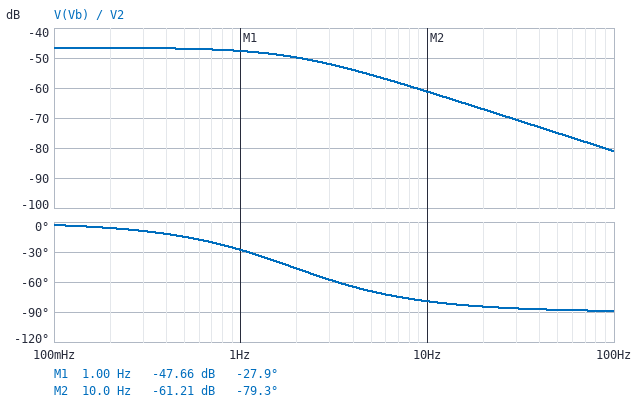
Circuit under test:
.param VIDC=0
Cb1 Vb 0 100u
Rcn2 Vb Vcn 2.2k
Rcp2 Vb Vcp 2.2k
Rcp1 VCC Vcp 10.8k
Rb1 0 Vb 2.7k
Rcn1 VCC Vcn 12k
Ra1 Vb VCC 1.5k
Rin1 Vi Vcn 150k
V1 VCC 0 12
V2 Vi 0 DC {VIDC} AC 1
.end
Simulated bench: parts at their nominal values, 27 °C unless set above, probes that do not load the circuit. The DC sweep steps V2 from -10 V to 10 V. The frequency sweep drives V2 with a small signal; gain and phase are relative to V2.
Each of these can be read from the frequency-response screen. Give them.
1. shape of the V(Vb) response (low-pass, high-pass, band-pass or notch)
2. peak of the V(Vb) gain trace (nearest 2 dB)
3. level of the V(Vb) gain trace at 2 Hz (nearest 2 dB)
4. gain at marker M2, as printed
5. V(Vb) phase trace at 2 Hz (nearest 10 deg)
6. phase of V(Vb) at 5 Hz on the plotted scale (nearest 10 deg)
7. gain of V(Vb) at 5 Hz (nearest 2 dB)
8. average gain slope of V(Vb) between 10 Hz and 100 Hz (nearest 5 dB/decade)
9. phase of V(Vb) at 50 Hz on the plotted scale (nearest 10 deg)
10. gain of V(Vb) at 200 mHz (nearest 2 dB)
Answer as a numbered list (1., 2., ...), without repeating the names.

1. low-pass
2. -46 dB
3. -50 dB
4. -61.21 dB
5. -50 deg
6. -70 deg
7. -56 dB
8. -20 dB/decade
9. -90 deg
10. -46 dB
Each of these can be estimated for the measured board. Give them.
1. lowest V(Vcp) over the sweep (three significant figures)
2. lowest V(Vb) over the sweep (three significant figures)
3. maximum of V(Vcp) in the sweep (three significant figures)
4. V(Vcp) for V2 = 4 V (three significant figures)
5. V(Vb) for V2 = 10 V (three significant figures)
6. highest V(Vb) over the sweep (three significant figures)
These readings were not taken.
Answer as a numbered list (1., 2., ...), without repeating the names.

1. 8.81 V
2. 8.16 V
3. 8.89 V
4. 8.86 V
5. 8.25 V
6. 8.25 V
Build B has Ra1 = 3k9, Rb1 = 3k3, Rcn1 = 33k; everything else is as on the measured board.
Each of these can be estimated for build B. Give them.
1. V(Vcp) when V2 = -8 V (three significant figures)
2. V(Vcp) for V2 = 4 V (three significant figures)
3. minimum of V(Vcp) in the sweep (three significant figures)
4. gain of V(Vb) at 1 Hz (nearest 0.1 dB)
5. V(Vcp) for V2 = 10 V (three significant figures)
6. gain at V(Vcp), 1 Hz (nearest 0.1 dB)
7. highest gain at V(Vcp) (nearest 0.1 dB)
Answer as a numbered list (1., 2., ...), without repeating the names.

1. 7.34 V
2. 7.43 V
3. 7.33 V
4. -43.5 dB
5. 7.48 V
6. -45.1 dB
7. -42.3 dB
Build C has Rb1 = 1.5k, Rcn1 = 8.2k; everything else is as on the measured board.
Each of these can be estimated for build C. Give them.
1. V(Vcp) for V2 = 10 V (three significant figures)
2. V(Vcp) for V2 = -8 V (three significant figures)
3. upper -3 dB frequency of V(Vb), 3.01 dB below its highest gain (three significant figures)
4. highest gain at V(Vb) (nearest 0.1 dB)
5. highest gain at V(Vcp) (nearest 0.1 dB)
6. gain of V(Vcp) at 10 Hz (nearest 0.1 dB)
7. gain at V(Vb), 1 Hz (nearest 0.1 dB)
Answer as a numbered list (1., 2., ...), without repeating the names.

1. 7.59 V
2. 7.54 V
3. 2.40 Hz
4. -49.3 dB
5. -50.9 dB
6. -63.5 dB
7. -50.0 dB
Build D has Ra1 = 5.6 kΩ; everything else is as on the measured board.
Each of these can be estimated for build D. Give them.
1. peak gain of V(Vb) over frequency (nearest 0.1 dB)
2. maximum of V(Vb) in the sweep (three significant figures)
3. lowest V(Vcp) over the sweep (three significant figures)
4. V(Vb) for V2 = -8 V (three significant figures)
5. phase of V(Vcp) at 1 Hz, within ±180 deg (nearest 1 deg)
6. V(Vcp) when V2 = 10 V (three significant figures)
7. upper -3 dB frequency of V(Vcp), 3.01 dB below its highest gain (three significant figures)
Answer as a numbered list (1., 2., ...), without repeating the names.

1. -42.0 dB
2. 5.64 V
3. 6.59 V
4. 5.50 V
5. -42 deg
6. 6.72 V
7. 1.12 Hz
